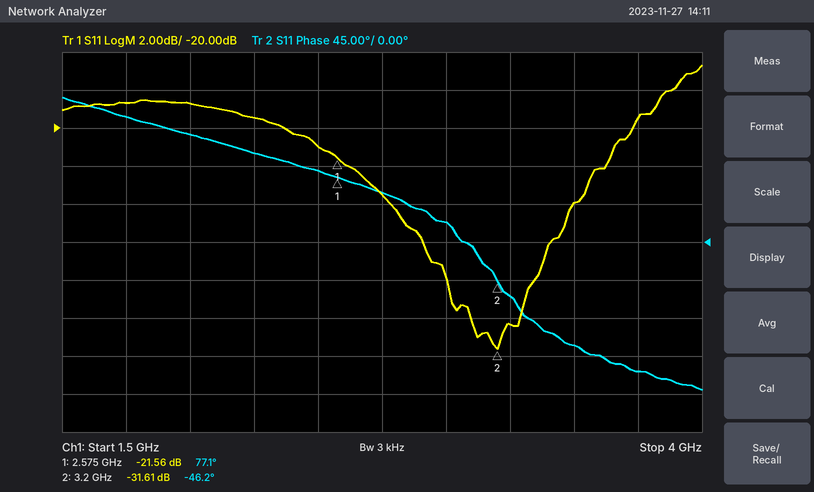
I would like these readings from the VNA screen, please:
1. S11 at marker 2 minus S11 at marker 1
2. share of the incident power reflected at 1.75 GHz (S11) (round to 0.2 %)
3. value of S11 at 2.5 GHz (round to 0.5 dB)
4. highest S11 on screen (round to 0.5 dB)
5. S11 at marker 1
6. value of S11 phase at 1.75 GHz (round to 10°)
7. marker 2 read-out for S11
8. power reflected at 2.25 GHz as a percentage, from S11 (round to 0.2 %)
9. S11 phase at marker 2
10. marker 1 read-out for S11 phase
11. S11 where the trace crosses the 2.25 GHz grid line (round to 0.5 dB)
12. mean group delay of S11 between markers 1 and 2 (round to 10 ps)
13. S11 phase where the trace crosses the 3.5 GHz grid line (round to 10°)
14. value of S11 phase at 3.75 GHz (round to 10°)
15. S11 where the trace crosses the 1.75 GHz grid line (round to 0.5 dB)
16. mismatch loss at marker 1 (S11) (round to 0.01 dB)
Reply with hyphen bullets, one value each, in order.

- -10.05 dB
- 1.4 %
- -21.0 dB
- -16.5 dB
- -21.56 dB
- 150°
- -31.61 dB
- 1.2 %
- -46.2°
- 77.1°
- -19.5 dB
- 550 ps
- -120°
- -150°
- -18.5 dB
- 0.03 dB
